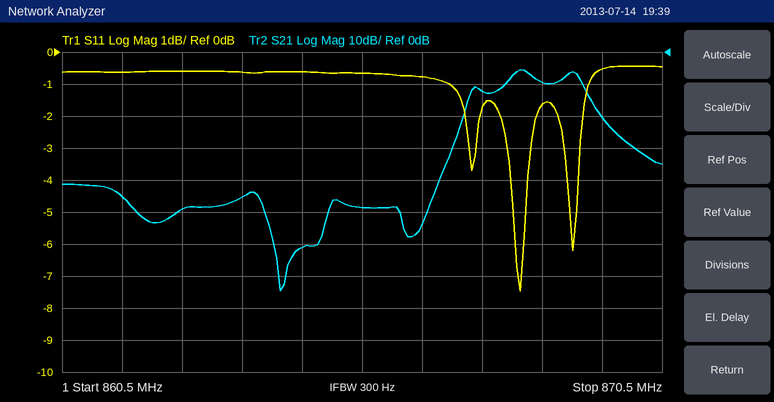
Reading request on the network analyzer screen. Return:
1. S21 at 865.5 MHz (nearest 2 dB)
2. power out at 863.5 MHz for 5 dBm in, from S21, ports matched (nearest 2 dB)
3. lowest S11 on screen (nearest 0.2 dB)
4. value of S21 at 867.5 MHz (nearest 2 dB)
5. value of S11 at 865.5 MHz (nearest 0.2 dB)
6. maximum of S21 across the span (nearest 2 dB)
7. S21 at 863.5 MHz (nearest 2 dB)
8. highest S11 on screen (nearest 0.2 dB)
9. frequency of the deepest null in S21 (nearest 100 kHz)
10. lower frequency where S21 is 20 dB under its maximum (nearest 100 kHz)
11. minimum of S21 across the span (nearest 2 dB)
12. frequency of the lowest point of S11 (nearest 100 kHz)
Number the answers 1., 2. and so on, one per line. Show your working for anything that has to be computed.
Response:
1. -48 dB
2. 5 dBm + (-46 dB) = -40 dBm
3. -7.4 dB
4. -12 dB
5. -0.6 dB
6. -6 dB
7. -46 dB
8. -0.4 dB
9. 864.1 MHz
10. 867.1 MHz
11. -74 dB
12. 868.1 MHz
